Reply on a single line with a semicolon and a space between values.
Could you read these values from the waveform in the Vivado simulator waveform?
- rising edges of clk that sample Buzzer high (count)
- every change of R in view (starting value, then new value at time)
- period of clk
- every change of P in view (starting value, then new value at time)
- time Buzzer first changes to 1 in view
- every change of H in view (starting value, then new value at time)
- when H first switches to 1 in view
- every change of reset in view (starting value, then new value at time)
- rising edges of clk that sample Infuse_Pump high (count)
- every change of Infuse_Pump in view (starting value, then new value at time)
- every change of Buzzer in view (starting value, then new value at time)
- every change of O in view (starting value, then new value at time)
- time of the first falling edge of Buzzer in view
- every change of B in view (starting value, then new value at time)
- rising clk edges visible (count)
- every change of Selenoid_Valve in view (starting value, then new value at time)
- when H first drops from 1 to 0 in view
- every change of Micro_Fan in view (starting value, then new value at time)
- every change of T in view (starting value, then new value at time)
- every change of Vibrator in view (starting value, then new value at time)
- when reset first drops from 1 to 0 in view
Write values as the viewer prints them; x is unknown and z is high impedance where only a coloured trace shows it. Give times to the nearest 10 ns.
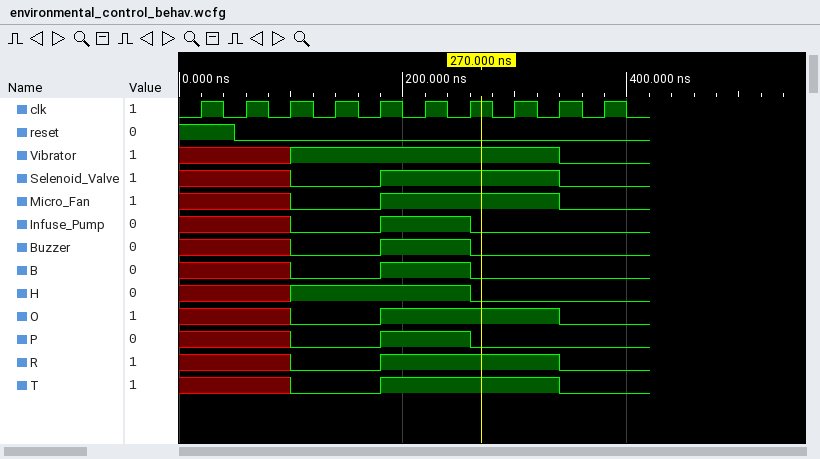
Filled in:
2; x, 0 at 100 ns, 1 at 180 ns, 0 at 340 ns; 40 ns; x, 0 at 100 ns, 1 at 180 ns, 0 at 260 ns; 180 ns; x, 1 at 100 ns, 0 at 260 ns; 100 ns; 1, 0 at 50 ns; 2; x, 0 at 100 ns, 1 at 180 ns, 0 at 260 ns; x, 0 at 100 ns, 1 at 180 ns, 0 at 260 ns; x, 0 at 100 ns, 1 at 180 ns, 0 at 340 ns; 260 ns; x, 0 at 100 ns, 1 at 180 ns, 0 at 260 ns; 10; x, 0 at 100 ns, 1 at 180 ns, 0 at 340 ns; 260 ns; x, 0 at 100 ns, 1 at 180 ns, 0 at 340 ns; x, 0 at 100 ns, 1 at 180 ns, 0 at 340 ns; x, 1 at 100 ns, 0 at 340 ns; 50 ns
